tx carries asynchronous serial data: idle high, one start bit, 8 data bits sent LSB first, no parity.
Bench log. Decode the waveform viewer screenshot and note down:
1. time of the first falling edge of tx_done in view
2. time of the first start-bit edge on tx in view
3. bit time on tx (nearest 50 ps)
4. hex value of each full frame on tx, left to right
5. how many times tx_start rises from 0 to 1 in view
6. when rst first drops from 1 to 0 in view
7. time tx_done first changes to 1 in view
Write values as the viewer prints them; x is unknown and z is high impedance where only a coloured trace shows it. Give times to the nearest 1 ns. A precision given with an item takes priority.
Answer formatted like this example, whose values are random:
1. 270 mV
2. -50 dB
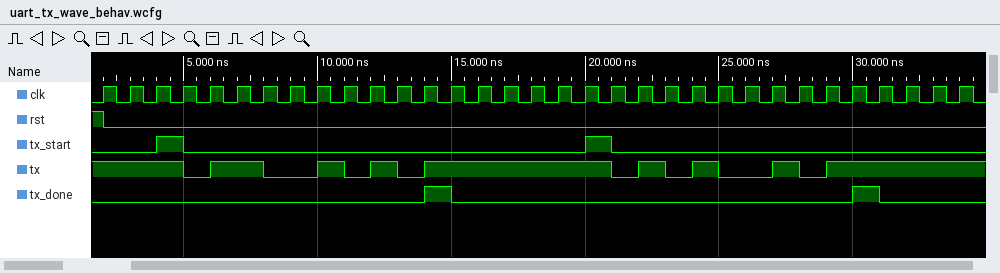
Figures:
1. 15 ns
2. 5 ns
3. 1000 ps
4. 53, A5
5. 2
6. 2 ns
7. 14 ns
